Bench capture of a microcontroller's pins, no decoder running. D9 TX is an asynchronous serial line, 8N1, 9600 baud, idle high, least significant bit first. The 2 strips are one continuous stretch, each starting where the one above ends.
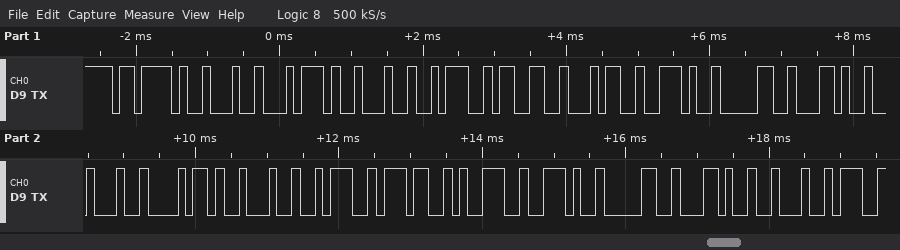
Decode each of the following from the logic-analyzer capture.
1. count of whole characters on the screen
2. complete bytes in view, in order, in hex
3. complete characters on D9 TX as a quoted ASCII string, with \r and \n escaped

20
0x7B 0x22 0x74 0x22 0x3A 0x33 0x34 0x2E 0x30 0x2C 0x22 0x68 0x22 0x3A 0x37 0x39 0x2E 0x30 0x2C 0x22
"{\"t\":34.0,\"h\":79.0,\""
